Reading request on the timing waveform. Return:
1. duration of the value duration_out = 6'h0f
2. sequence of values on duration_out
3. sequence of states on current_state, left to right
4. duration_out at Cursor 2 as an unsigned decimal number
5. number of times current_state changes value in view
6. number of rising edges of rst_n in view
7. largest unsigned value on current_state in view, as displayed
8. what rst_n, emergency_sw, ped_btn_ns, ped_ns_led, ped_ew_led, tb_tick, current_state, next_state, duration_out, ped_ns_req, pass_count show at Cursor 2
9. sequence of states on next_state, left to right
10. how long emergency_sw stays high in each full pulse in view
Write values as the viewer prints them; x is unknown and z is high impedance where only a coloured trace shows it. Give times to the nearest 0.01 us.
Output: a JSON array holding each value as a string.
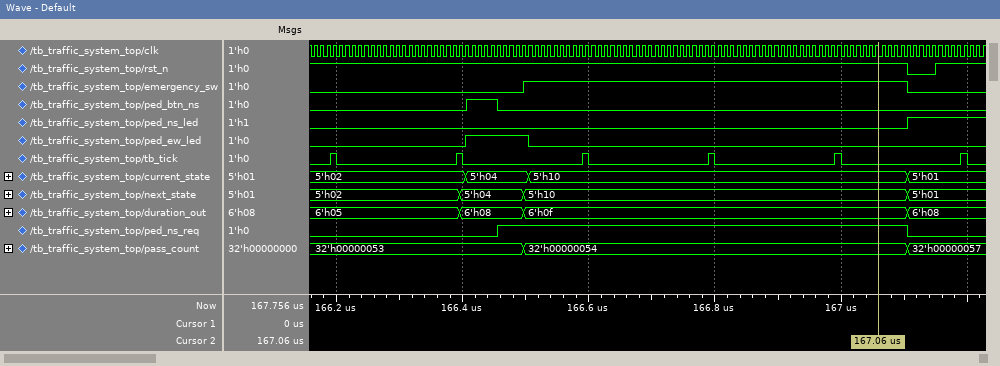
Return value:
["0.61 us", "6'h05, 6'h08, 6'h0f, 6'h08", "5'h02, 5'h04, 5'h10, 5'h01", "15", "3", "1", "5'h10", "rst_n=1, emergency_sw=1, ped_btn_ns=0, ped_ns_led=0, ped_ew_led=0, tb_tick=0, current_state=5'h10, next_state=5'h10, duration_out=6'h0f, ped_ns_req=1, pass_count=32'h00000054", "5'h02, 5'h04, 5'h10, 5'h01", "0.61 us"]
